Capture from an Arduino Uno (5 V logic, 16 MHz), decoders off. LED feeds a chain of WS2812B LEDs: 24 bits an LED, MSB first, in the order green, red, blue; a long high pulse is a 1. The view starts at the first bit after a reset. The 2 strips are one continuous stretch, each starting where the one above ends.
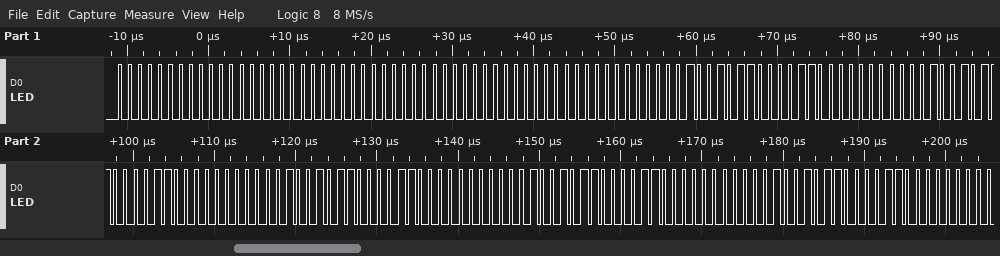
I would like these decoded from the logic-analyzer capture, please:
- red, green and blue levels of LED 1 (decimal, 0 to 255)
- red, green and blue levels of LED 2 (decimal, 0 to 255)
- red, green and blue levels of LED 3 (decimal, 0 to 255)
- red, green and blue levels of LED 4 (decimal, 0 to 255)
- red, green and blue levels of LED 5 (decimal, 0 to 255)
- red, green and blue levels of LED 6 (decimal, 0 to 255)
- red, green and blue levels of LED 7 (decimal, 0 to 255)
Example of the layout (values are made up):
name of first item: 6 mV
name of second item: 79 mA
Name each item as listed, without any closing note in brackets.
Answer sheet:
red, green and blue levels of LED 1: 0, 0, 0
red, green and blue levels of LED 2: 0, 0, 0
red, green and blue levels of LED 3: 150, 0, 24
red, green and blue levels of LED 4: 150, 0, 24
red, green and blue levels of LED 5: 150, 0, 24
red, green and blue levels of LED 6: 150, 0, 24
red, green and blue levels of LED 7: 150, 0, 24
